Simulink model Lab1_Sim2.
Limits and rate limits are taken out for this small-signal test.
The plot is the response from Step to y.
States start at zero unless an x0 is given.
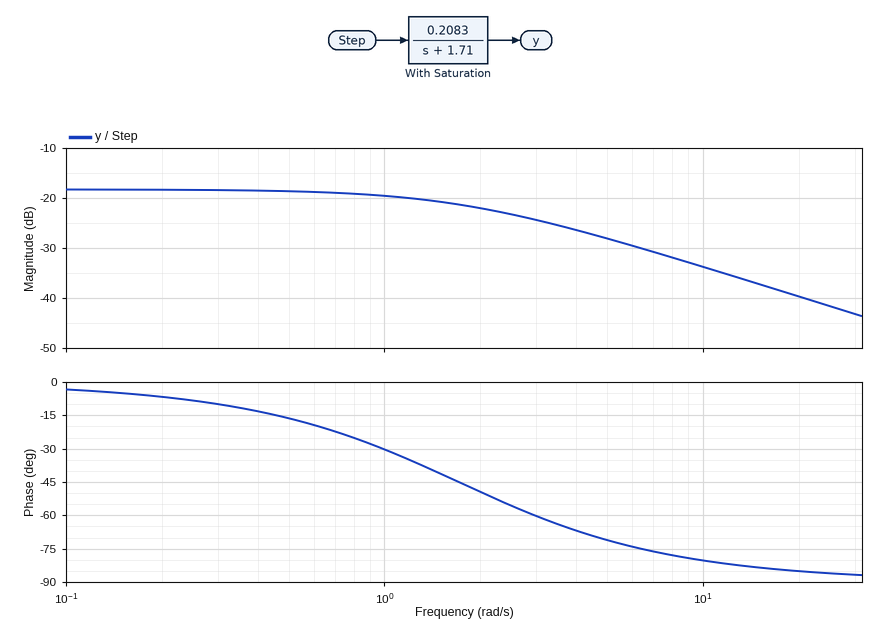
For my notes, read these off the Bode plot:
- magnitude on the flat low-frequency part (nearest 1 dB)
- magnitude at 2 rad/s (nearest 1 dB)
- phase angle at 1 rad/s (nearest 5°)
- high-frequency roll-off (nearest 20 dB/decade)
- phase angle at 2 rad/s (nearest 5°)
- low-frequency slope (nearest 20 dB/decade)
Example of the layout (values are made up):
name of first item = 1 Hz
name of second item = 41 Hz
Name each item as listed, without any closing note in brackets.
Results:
magnitude on the flat low-frequency part = -18 dB
magnitude at 2 rad/s = -22 dB
phase angle at 1 rad/s = -30°
high-frequency roll-off = -20 dB/decade
phase angle at 2 rad/s = -50°
low-frequency slope = 0 dB/decade
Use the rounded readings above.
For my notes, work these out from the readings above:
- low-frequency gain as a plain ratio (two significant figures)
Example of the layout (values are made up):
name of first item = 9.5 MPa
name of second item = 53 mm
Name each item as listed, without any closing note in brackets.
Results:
low-frequency gain as a plain ratio = 0.13
